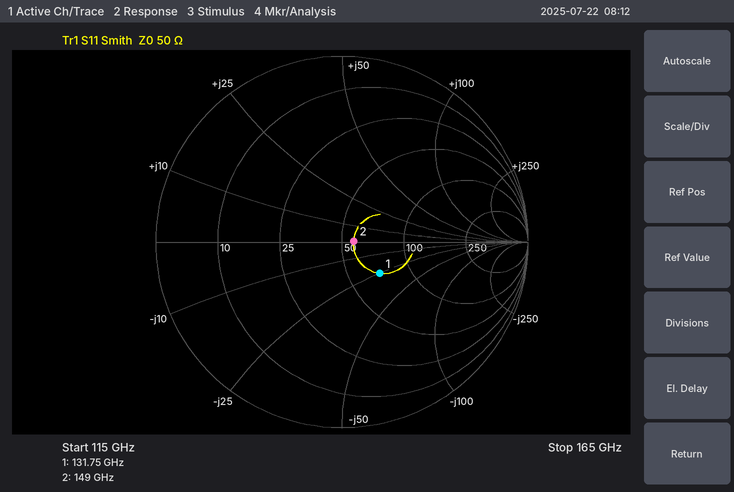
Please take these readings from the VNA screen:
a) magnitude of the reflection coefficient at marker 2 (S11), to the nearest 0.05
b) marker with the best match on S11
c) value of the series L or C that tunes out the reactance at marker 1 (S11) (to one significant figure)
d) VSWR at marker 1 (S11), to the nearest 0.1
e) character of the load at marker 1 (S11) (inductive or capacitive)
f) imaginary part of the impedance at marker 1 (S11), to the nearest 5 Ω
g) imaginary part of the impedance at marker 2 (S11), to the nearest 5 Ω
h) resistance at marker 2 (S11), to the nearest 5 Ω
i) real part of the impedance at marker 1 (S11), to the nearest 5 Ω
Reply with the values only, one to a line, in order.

0.05
marker 2
30 pH
1.7
capacitive
-25 Ω
0 Ω
55 Ω
70 Ω
